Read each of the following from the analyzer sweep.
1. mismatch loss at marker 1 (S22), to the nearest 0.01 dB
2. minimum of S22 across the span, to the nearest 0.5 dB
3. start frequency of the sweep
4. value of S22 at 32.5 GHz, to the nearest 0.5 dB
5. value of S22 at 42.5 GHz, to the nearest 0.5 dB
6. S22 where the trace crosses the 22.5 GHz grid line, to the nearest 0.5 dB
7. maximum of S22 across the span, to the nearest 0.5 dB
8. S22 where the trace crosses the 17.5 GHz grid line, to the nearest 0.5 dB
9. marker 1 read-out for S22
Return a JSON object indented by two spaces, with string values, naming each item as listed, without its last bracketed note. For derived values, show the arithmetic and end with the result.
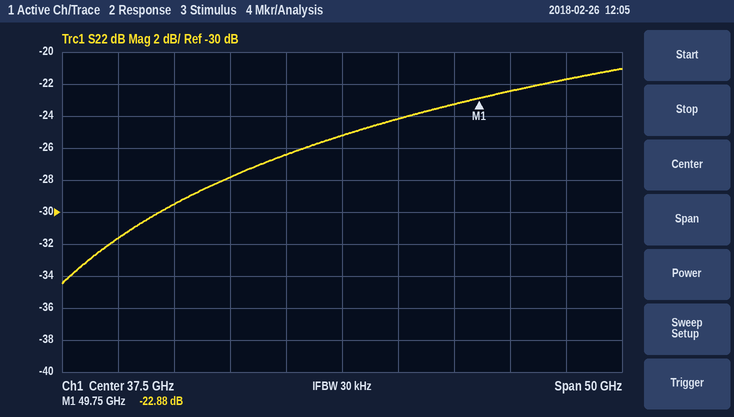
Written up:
{
  "mismatch loss at marker 1 (S22), to the nearest 0.01 dB": "−10 log10(1 − 10^(-22.88/10)) ≈ 0.02 dB",
  "minimum of S22 across the span, to the nearest 0.5 dB": "-34.5 dB",
  "start frequency of the sweep": "12.5 GHz",
  "value of S22 at 32.5 GHz, to the nearest 0.5 dB": "-26.5 dB",
  "value of S22 at 42.5 GHz, to the nearest 0.5 dB": "-24.0 dB",
  "S22 where the trace crosses the 22.5 GHz grid line, to the nearest 0.5 dB": "-29.5 dB",
  "maximum of S22 across the span, to the nearest 0.5 dB": "-21.0 dB",
  "S22 where the trace crosses the 17.5 GHz grid line, to the nearest 0.5 dB": "-31.5 dB",
  "marker 1 read-out for S22": "-22.88 dB"
}
